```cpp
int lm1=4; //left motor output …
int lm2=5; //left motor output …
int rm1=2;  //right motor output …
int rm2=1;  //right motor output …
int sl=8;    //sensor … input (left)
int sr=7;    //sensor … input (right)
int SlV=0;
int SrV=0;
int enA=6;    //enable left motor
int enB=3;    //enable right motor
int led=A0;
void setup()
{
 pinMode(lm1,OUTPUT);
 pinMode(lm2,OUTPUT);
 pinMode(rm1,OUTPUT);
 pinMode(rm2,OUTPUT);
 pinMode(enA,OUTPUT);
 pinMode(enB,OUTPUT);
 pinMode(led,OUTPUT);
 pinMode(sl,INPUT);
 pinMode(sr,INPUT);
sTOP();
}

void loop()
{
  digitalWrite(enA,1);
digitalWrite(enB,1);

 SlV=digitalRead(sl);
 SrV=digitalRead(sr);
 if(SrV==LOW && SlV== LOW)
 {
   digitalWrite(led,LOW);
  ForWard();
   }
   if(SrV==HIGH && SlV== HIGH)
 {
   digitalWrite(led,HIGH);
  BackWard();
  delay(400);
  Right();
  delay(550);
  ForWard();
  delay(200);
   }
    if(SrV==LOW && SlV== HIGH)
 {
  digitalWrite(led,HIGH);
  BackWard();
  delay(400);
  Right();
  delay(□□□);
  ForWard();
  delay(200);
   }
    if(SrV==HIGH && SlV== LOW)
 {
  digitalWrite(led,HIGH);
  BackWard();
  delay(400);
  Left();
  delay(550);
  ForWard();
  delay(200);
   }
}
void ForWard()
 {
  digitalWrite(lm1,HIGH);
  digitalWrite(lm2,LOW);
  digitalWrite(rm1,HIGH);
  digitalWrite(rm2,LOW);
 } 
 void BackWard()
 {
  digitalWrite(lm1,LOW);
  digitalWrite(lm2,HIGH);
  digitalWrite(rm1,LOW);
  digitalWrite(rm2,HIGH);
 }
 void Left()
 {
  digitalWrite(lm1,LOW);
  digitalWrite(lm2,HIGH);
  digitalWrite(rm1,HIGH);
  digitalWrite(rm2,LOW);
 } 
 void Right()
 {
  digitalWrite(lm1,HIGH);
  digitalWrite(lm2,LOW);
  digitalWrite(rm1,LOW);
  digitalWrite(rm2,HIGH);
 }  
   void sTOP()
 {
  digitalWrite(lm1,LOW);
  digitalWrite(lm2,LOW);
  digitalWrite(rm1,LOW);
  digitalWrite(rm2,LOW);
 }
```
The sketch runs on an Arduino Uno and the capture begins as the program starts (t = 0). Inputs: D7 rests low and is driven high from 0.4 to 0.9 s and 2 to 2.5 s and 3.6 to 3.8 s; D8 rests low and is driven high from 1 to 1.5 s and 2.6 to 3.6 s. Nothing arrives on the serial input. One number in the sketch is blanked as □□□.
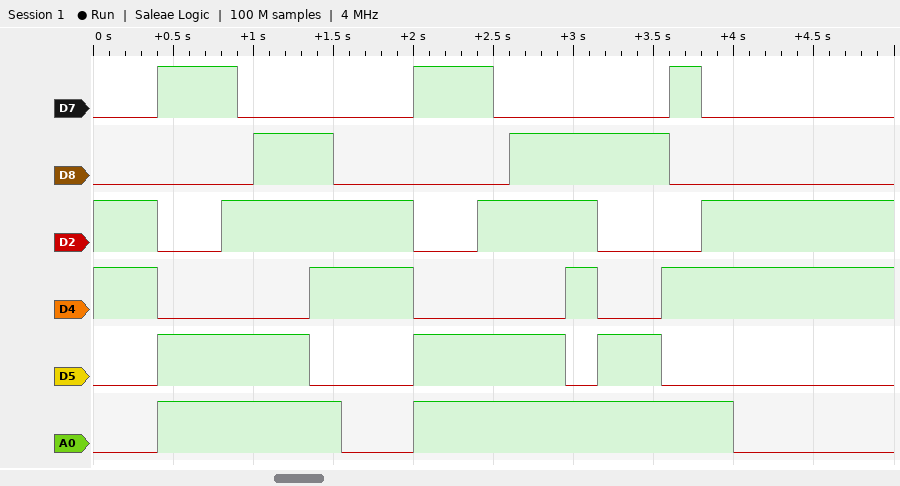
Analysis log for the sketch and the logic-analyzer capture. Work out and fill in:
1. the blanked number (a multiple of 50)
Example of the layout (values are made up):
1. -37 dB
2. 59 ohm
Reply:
1. 250
